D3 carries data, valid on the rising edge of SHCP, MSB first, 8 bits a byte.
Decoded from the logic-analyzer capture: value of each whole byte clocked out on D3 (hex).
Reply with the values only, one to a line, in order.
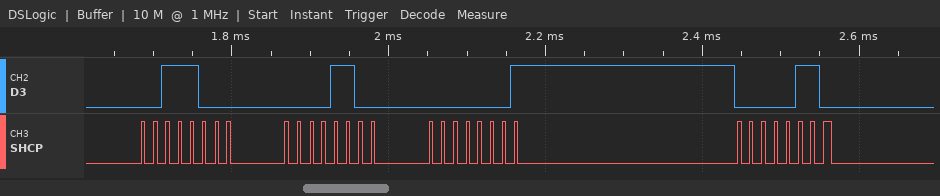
38 0C 01 06
